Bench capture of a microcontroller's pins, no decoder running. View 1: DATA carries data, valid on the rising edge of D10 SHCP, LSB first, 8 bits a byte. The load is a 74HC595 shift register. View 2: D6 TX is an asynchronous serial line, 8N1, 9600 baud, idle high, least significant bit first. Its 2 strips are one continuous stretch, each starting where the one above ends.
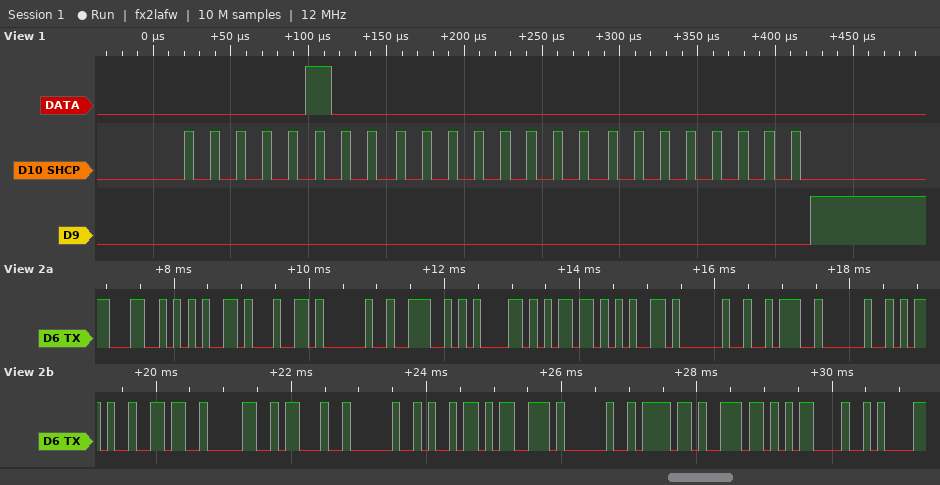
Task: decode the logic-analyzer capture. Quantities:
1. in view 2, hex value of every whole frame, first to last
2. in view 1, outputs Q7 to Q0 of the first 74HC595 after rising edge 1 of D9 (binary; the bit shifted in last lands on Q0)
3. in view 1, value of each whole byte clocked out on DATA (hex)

4C 65 64 20 4E 61 6D 65 20 3A 20 2D 36 30 23 20 69 73 20 6F 6E 0D 0A
00000000
20 00 00
